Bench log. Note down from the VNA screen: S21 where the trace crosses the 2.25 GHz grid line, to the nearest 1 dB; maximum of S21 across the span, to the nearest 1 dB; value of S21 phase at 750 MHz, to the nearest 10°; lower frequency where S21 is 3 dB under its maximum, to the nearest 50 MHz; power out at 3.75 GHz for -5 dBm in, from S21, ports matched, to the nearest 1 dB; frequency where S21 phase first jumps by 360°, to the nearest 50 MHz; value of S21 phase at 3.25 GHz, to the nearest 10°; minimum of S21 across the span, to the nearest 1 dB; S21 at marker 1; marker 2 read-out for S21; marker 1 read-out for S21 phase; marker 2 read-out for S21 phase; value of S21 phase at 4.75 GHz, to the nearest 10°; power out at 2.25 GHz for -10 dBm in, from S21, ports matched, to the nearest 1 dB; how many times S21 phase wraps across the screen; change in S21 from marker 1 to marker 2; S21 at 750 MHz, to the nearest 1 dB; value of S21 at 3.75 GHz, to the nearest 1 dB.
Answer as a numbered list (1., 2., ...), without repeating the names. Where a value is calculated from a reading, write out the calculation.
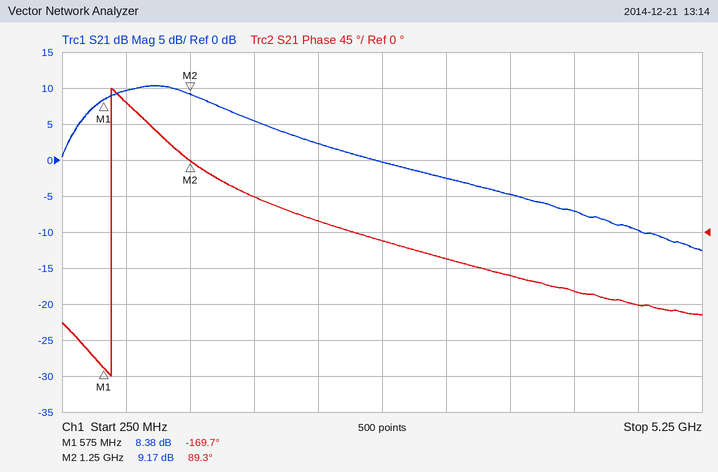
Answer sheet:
1. 2 dB
2. 10 dB
3. 160°
4. 500 MHz
5. -5 dBm + (-5 dB) = -10 dBm
6. 650 MHz
7. -30°
8. -13 dB
9. 8.38 dB
10. 9.17 dB
11. -169.7°
12. 89.3°
13. -90°
14. -10 dBm + (2 dB) = -8 dBm
15. 1
16. 9.17 − (8.38) = 0.79 dB
17. 10 dB
18. -5 dB
